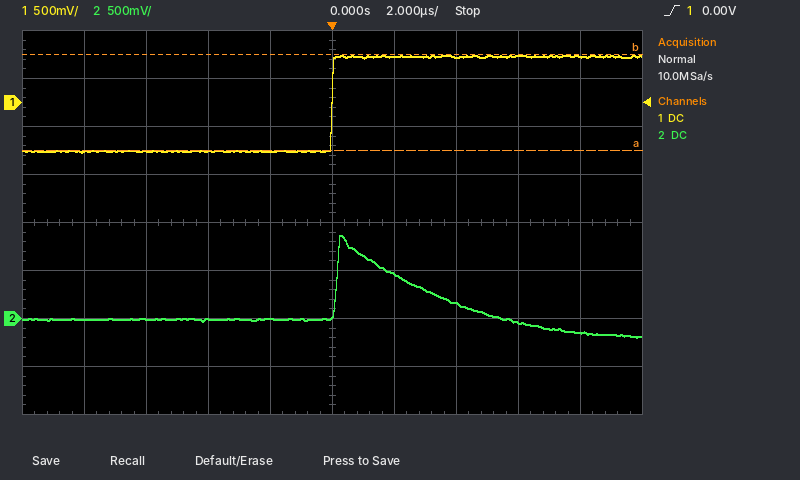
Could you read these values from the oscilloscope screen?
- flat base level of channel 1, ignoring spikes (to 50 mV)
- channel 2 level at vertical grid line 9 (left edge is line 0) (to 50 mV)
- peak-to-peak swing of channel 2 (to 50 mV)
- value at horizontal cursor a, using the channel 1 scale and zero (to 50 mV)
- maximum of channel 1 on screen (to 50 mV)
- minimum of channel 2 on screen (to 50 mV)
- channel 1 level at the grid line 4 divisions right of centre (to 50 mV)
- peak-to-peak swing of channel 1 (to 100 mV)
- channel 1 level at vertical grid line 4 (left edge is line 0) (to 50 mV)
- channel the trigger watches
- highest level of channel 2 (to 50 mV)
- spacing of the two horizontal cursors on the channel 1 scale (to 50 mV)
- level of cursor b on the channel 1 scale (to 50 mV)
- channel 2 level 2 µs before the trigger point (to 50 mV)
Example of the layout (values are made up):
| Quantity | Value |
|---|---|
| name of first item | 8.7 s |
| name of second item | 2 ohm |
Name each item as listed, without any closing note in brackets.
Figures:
| Quantity | Value |
|---|---|
| flat base level of channel 1, ignoring spikes | -500 mV |
| channel 2 level at vertical grid line 9 (left edge is line 0) | -150 mV |
| peak-to-peak swing of channel 2 | 1.05 V |
| value at horizontal cursor a, using the channel 1 scale and zero | -500 mV |
| maximum of channel 1 on screen | 500 mV |
| minimum of channel 2 on screen | -200 mV |
| channel 1 level at the grid line 4 divisions right of centre | 500 mV |
| peak-to-peak swing of channel 1 | 1.00 V |
| channel 1 level at vertical grid line 4 (left edge is line 0) | -500 mV |
| channel the trigger watches | channel 1 |
| highest level of channel 2 | 850 mV |
| spacing of the two horizontal cursors on the channel 1 scale | 1.00 V |
| level of cursor b on the channel 1 scale | 500 mV |
| channel 2 level 2 µs before the trigger point | 0 mV |
